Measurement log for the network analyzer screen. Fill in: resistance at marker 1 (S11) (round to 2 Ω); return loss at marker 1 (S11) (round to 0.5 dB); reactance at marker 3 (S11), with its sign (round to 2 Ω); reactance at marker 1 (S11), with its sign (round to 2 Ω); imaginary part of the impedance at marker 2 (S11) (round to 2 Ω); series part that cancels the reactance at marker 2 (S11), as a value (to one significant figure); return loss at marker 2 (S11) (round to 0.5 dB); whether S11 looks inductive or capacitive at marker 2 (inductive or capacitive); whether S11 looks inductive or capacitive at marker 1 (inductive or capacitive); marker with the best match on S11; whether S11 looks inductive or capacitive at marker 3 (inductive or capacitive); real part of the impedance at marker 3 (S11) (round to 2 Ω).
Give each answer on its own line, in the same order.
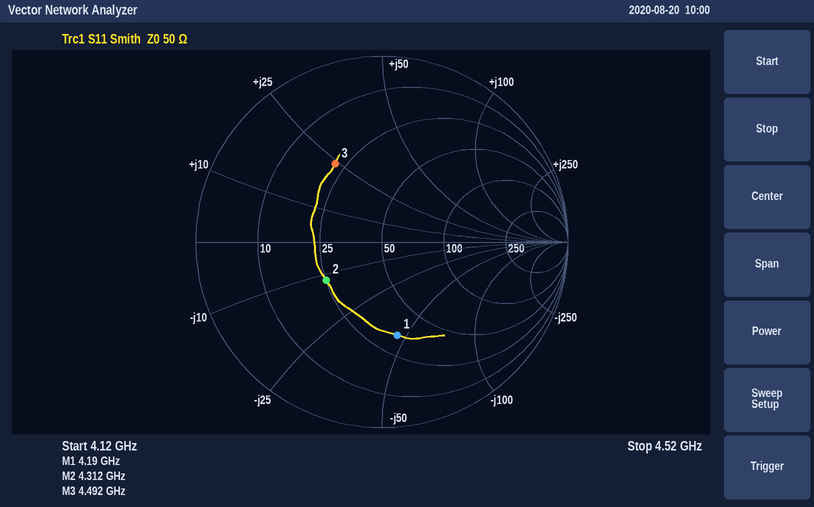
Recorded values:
34 Ω
6.0 dB
+24 Ω
-46 Ω
-12 Ω
400 pH
9.0 dB
capacitive
capacitive
marker 2
inductive
22 Ω
